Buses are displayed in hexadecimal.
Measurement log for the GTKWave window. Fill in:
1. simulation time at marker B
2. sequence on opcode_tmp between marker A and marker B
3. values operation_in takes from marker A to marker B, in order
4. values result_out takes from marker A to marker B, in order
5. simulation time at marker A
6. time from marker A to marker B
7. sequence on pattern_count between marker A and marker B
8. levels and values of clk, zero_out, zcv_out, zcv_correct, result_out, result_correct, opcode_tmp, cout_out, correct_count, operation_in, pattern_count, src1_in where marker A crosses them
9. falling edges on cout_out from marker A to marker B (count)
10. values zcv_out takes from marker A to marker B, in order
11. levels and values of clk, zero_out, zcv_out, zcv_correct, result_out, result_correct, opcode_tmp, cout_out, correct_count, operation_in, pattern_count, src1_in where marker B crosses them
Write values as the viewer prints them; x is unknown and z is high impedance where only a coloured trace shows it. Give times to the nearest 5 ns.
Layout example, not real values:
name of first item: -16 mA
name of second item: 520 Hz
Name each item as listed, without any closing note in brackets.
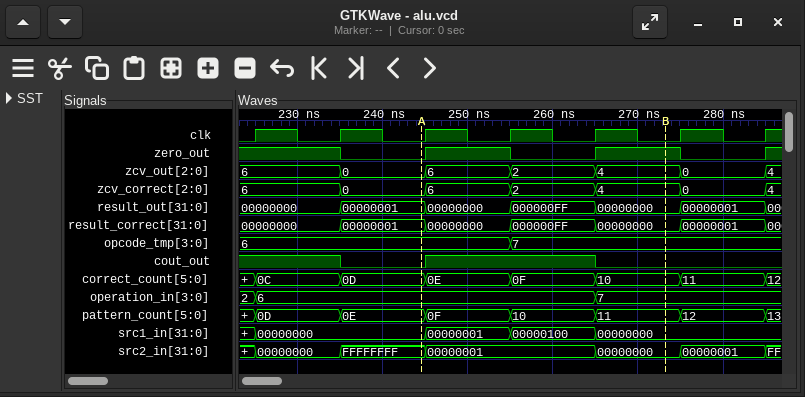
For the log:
simulation time at marker B: 275 ns
sequence on opcode_tmp between marker A and marker B: 6, 7
values operation_in takes from marker A to marker B, in order: 6, 7
values result_out takes from marker A to marker B, in order: 00000001, 00000000, 000000FF, 00000000
simulation time at marker A: 245 ns
time from marker A to marker B: 30 ns
sequence on pattern_count between marker A and marker B: 0E, 0F, 10, 11
levels and values of clk, zero_out, zcv_out, zcv_correct, result_out, result_correct, opcode_tmp, cout_out, correct_count, operation_in, pattern_count, src1_in where marker A crosses them: clk=0, zero_out=0, zcv_out=0, zcv_correct=0, result_out=00000001, result_correct=00000001, opcode_tmp=6, cout_out=0, correct_count=0D, operation_in=6, pattern_count=0E, src1_in=00000000
falling edges on cout_out from marker A to marker B: 1
values zcv_out takes from marker A to marker B, in order: 0, 6, 2, 4
levels and values of clk, zero_out, zcv_out, zcv_correct, result_out, result_correct, opcode_tmp, cout_out, correct_count, operation_in, pattern_count, src1_in where marker B crosses them: clk=0, zero_out=1, zcv_out=4, zcv_correct=4, result_out=00000000, result_correct=00000000, opcode_tmp=7, cout_out=0, correct_count=10, operation_in=7, pattern_count=11, src1_in=00000000
